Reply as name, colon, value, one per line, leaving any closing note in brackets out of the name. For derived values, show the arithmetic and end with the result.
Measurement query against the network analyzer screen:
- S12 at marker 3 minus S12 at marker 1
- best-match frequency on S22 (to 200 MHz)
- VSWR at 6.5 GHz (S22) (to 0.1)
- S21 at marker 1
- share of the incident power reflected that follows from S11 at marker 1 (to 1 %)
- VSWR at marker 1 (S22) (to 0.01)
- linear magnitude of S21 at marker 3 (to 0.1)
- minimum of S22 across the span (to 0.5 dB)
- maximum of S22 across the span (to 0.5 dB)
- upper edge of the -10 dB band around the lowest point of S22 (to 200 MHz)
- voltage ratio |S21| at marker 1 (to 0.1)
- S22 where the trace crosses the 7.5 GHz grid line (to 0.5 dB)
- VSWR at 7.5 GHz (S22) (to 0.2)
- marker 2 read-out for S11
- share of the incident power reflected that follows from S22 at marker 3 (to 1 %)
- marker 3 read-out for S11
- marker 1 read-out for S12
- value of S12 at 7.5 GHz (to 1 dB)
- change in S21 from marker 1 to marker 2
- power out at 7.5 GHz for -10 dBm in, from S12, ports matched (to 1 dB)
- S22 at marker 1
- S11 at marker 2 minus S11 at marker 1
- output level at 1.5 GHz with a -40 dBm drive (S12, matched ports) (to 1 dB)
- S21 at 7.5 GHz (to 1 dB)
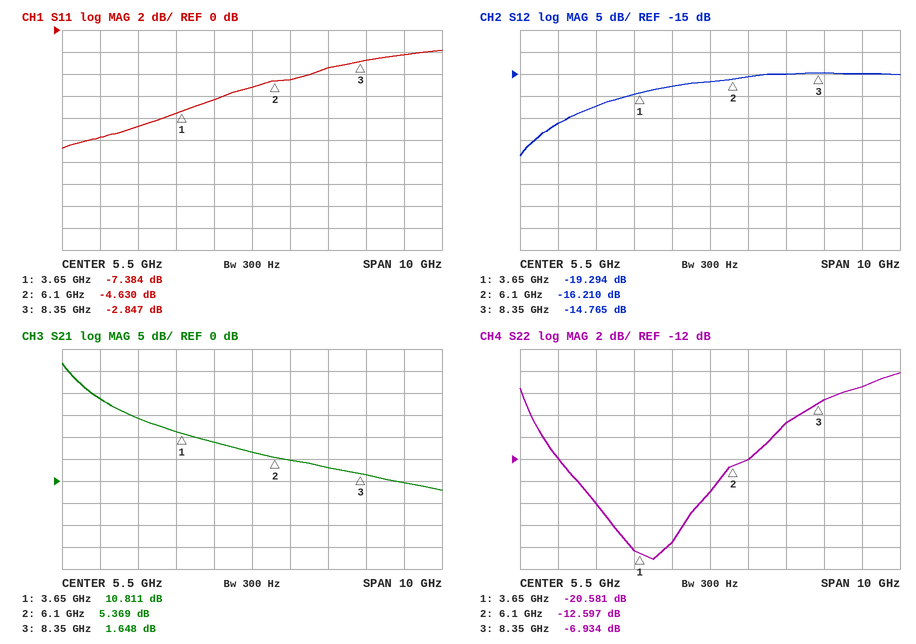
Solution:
S12 at marker 3 minus S12 at marker 1: -14.765 − (-19.294) = 4.529 dB
best-match frequency on S22: 4.0 GHz
VSWR at 6.5 GHz (S22): |Γ| = 10^(-12/20) = 0.2512; VSWR = (1 + 0.2512)/(1 − 0.2512) ≈ 1.7
S21 at marker 1: 10.811 dB
share of the incident power reflected that follows from S11 at marker 1: 10^(-7.384/10) ≈ 18 %
VSWR at marker 1 (S22): (1 + 0.0935)/(1 − 0.0935) ≈ 1.21
linear magnitude of S21 at marker 3: 10^(1.648/20) ≈ 1.2
minimum of S22 across the span: -21.0 dB
maximum of S22 across the span: -4.0 dB
upper edge of the -10 dB band around the lowest point of S22: 7.2 GHz
voltage ratio |S21| at marker 1: 10^(10.811/20) ≈ 3.5
S22 where the trace crosses the 7.5 GHz grid line: -8.5 dB
VSWR at 7.5 GHz (S22): |Γ| = 10^(-8.5/20) = 0.3758; VSWR = (1 + 0.3758)/(1 − 0.3758) ≈ 2.2
marker 2 read-out for S11: -4.630 dB
share of the incident power reflected that follows from S22 at marker 3: 10^(-6.934/10) ≈ 20 %
marker 3 read-out for S11: -2.847 dB
marker 1 read-out for S12: -19.294 dB
value of S12 at 7.5 GHz: -15 dB
change in S21 from marker 1 to marker 2: 5.369 − (10.811) = -5.442 dB
power out at 7.5 GHz for -10 dBm in, from S12, ports matched: -10 dBm + (-15 dB) = -25 dBm
S22 at marker 1: -20.581 dB
S11 at marker 2 minus S11 at marker 1: -4.63 − (-7.384) = 2.754 dB
output level at 1.5 GHz with a -40 dBm drive (S12, matched ports): -40 dBm + (-26 dB) = -66 dBm
S21 at 7.5 GHz: 3 dB
